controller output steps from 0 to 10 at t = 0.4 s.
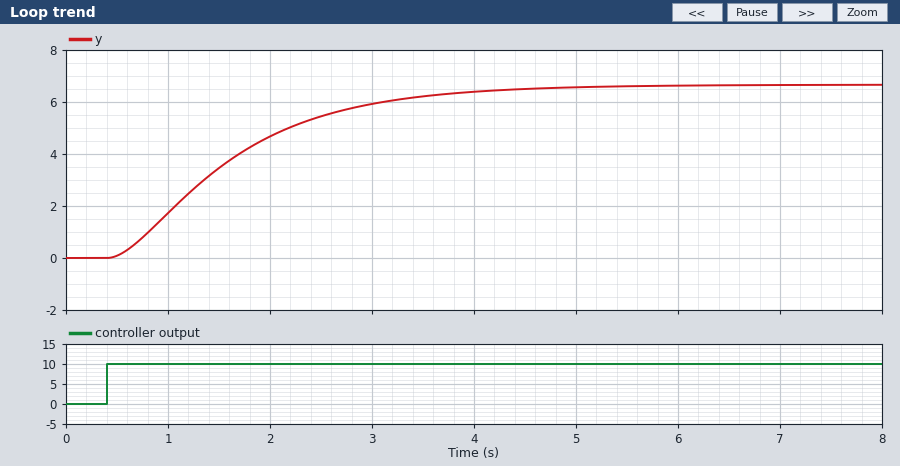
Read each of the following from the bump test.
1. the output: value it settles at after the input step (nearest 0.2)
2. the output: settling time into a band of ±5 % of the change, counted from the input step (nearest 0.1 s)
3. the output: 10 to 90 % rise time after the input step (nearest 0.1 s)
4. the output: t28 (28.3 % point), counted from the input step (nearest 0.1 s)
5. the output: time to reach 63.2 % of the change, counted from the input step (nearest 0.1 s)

6.6
3.4 s
2.4 s
0.6 s
1.4 s
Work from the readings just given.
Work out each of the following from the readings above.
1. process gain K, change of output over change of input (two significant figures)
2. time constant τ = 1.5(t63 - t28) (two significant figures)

0.66
1.2 s
